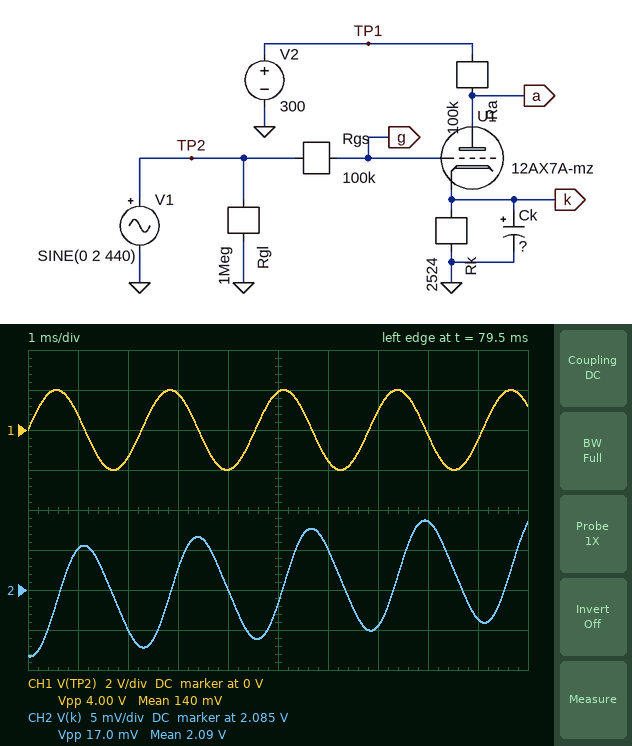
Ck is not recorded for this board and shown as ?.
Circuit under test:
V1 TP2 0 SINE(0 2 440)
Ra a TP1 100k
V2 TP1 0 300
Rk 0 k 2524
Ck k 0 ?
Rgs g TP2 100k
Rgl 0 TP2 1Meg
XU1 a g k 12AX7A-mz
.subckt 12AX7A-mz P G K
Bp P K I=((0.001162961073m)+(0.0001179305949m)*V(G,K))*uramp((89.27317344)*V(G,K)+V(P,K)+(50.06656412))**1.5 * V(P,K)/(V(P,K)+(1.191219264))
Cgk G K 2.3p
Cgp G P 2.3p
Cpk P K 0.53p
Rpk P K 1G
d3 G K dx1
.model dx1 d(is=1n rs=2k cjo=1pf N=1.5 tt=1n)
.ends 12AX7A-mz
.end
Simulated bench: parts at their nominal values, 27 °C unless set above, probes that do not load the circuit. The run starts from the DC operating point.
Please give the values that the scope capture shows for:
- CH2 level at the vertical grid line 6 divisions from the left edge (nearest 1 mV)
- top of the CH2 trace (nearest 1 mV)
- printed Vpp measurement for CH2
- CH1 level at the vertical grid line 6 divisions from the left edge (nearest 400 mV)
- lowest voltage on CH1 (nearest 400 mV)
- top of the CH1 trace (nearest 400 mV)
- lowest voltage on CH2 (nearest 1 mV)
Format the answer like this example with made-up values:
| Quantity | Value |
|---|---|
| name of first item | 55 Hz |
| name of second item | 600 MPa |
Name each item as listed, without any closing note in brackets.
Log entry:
| Quantity | Value |
|---|---|
| CH2 level at the vertical grid line 6 divisions from the left edge | 2.090 V |
| top of the CH2 trace | 2.094 V |
| printed Vpp measurement for CH2 | 17.0 mV |
| CH1 level at the vertical grid line 6 divisions from the left edge | -1.6 V |
| lowest voltage on CH1 | -2.0 V |
| top of the CH1 trace | 2.0 V |
| lowest voltage on CH2 | 2.077 V |
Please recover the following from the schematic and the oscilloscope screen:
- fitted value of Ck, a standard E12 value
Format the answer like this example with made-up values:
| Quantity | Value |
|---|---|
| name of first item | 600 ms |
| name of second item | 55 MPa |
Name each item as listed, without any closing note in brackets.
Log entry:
| Quantity | Value |
|---|---|
| fitted value of Ck, a standard E12 value | 56 µF |
